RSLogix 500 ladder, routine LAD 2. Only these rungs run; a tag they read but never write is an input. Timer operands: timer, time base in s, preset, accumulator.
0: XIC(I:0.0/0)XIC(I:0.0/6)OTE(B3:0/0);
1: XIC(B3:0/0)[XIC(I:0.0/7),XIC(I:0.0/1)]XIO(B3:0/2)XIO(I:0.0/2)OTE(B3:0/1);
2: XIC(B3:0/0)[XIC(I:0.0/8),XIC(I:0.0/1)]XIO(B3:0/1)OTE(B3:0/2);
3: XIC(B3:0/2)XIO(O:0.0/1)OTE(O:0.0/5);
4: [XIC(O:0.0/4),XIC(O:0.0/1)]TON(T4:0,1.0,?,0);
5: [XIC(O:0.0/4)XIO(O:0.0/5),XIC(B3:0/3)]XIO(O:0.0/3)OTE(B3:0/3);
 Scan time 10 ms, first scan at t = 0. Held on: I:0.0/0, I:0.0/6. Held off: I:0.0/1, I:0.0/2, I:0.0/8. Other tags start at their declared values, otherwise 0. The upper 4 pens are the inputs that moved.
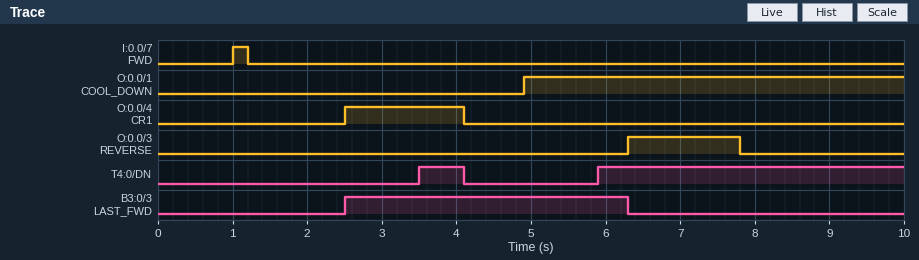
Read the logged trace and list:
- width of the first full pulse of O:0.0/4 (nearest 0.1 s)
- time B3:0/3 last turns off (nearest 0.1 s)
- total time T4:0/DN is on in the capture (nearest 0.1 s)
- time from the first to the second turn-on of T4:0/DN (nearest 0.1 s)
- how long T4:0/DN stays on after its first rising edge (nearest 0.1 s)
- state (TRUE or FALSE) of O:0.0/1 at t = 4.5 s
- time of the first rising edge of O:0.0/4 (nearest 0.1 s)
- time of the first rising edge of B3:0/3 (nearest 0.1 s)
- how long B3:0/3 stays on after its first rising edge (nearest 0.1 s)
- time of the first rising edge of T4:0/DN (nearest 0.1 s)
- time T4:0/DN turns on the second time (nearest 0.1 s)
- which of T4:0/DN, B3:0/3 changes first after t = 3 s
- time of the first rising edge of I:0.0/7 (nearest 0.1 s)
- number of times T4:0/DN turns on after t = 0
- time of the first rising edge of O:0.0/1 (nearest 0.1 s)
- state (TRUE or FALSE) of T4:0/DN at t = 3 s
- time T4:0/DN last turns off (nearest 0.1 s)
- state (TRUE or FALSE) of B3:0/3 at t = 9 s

1.6 s
6.3 s
4.7 s
2.4 s
0.6 s
FALSE
2.5 s
2.5 s
3.8 s
3.5 s
5.9 s
T4:0/DN
1.0 s
2
4.9 s
FALSE
4.1 s
FALSE
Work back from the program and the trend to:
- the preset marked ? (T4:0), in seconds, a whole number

1 s
